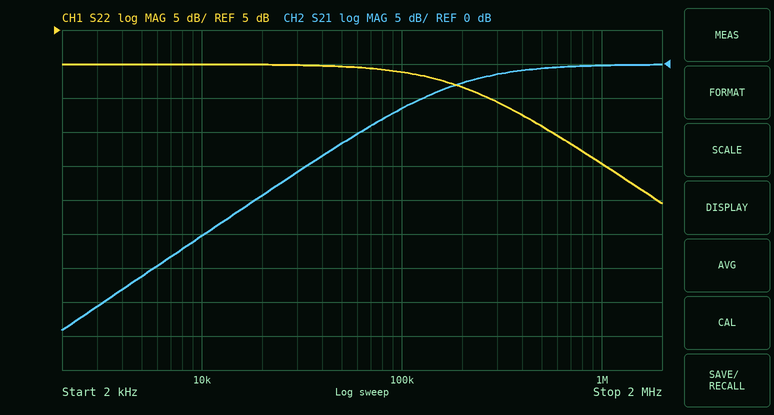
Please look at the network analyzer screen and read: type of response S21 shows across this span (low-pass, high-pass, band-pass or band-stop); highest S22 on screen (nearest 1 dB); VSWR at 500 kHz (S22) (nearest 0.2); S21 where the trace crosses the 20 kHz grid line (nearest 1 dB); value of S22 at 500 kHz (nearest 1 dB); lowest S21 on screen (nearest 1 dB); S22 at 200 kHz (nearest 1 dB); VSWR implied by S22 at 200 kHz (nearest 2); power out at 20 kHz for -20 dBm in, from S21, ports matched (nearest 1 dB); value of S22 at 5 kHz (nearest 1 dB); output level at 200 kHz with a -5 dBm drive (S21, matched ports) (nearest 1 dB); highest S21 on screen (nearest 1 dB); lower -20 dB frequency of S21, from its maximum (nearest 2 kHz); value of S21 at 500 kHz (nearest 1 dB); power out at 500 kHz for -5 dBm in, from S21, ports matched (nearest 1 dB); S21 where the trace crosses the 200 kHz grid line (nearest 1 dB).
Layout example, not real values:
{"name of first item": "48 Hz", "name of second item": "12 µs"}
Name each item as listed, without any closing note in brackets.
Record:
{"type of response S21 shows across this span": "high-pass", "highest S22 on screen": "0 dB", "VSWR at 500 kHz (S22)": "2.0", "S21 where the trace crosses the 20 kHz grid line": "-19 dB", "value of S22 at 500 kHz": "-9 dB", "lowest S21 on screen": "-39 dB", "S22 at 200 kHz": "-3 dB", "VSWR implied by S22 at 200 kHz": "6", "power out at 20 kHz for -20 dBm in, from S21, ports matched": "-39 dBm", "value of S22 at 5 kHz": "0 dB", "output level at 200 kHz with a -5 dBm drive (S21, matched ports)": "-8 dBm", "highest S21 on screen": "0 dB", "lower -20 dB frequency of S21, from its maximum": "18 kHz", "value of S21 at 500 kHz": "-1 dB", "power out at 500 kHz for -5 dBm in, from S21, ports matched": "-6 dBm", "S21 where the trace crosses the 200 kHz grid line": "-3 dB"}
